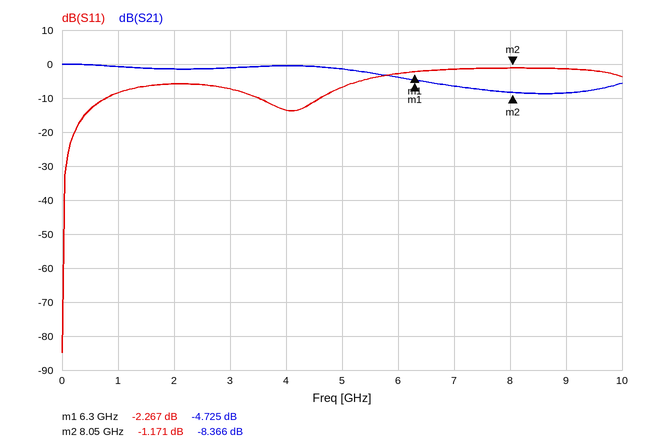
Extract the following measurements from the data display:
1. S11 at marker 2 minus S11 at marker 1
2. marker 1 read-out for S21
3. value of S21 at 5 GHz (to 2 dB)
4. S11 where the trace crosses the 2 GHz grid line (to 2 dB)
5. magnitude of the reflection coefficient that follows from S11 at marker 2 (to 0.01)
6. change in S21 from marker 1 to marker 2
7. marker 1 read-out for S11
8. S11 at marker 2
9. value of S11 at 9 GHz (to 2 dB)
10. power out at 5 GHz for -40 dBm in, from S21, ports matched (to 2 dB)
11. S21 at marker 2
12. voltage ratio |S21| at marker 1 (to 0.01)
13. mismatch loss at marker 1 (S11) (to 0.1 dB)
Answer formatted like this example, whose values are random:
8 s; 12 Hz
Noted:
1.096 dB; -4.725 dB; -2 dB; -6 dB; 0.87; -3.641 dB; -2.267 dB; -1.171 dB; -2 dB; -42 dBm; -8.366 dB; 0.58; 3.9 dB
